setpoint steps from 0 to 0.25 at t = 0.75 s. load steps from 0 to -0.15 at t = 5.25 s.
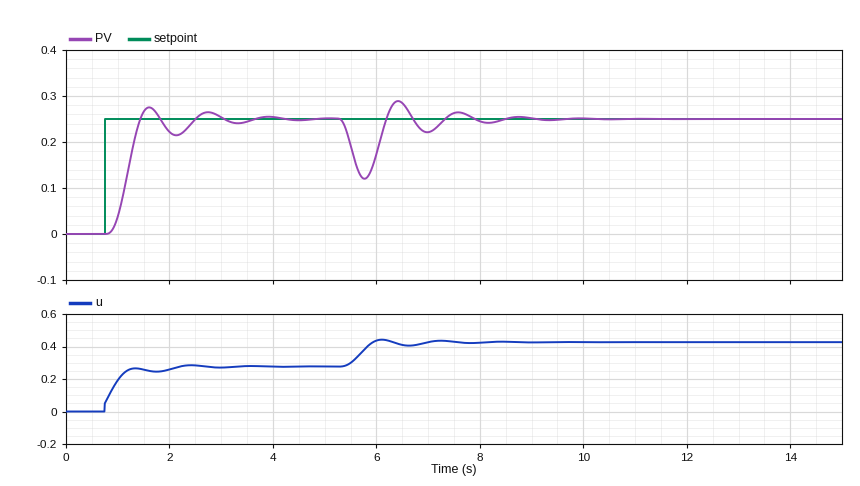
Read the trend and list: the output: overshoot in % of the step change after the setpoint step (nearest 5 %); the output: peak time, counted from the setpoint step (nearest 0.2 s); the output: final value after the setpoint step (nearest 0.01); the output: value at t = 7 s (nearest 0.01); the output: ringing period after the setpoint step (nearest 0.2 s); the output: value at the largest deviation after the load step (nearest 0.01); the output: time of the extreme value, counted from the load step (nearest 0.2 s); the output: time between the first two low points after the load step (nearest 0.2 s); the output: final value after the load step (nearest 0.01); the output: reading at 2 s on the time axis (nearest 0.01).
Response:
10 %
0.8 s
0.25
0.22
1.2 s
0.12
0.6 s
1.2 s
0.25
0.22
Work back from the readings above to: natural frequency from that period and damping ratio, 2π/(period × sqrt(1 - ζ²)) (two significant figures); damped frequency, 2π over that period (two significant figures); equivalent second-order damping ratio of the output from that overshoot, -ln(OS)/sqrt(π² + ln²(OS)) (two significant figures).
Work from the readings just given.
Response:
6.5 rad/s
5.2 rad/s
0.59
